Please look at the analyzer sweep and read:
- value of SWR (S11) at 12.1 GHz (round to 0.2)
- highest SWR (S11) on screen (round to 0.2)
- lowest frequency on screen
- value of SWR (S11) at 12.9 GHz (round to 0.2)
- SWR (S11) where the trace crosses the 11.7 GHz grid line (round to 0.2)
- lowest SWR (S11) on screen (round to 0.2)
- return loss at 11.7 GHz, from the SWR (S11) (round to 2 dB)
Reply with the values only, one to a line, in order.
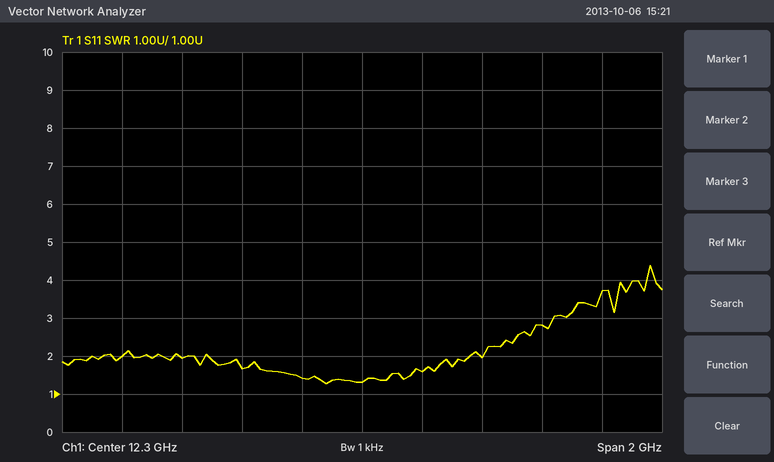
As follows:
1.4
4.4
11.3 GHz
2.8
2.0
1.2
10 dB
